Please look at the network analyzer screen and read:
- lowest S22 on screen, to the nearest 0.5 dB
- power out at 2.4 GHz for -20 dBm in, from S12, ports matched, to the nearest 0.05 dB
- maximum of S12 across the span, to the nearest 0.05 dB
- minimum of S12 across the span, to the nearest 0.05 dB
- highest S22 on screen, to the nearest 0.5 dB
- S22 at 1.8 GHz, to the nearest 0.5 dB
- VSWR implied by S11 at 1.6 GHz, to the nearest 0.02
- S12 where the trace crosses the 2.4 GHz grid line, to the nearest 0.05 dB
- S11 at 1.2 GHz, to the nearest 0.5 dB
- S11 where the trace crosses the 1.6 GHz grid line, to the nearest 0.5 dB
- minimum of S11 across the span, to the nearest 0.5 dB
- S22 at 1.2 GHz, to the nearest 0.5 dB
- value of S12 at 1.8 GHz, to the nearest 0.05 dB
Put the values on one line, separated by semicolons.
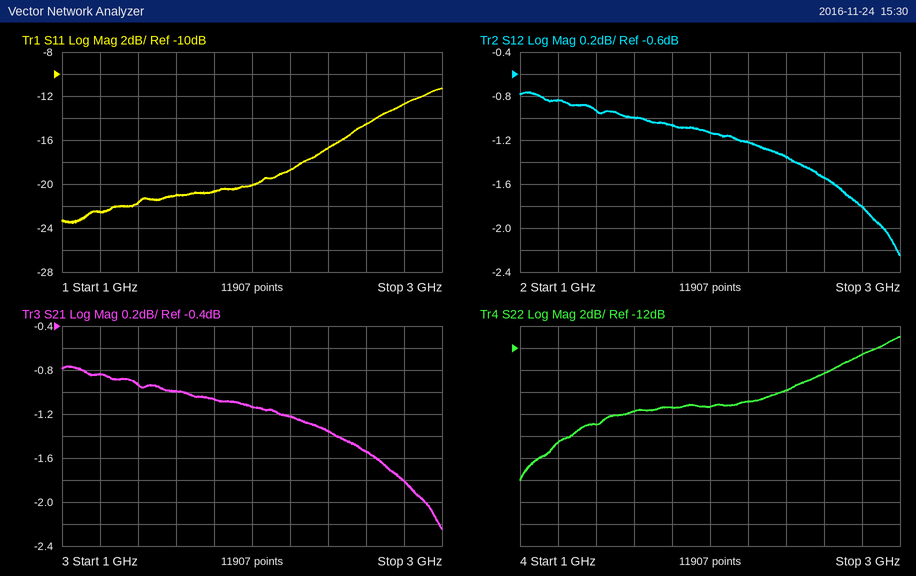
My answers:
-24.0 dB; -21.35 dBm; -0.75 dB; -2.25 dB; -11.0 dB; -17.5 dB; 1.20; -1.35 dB; -22.5 dB; -21.0 dB; -23.5 dB; -20.5 dB; -1.05 dB
